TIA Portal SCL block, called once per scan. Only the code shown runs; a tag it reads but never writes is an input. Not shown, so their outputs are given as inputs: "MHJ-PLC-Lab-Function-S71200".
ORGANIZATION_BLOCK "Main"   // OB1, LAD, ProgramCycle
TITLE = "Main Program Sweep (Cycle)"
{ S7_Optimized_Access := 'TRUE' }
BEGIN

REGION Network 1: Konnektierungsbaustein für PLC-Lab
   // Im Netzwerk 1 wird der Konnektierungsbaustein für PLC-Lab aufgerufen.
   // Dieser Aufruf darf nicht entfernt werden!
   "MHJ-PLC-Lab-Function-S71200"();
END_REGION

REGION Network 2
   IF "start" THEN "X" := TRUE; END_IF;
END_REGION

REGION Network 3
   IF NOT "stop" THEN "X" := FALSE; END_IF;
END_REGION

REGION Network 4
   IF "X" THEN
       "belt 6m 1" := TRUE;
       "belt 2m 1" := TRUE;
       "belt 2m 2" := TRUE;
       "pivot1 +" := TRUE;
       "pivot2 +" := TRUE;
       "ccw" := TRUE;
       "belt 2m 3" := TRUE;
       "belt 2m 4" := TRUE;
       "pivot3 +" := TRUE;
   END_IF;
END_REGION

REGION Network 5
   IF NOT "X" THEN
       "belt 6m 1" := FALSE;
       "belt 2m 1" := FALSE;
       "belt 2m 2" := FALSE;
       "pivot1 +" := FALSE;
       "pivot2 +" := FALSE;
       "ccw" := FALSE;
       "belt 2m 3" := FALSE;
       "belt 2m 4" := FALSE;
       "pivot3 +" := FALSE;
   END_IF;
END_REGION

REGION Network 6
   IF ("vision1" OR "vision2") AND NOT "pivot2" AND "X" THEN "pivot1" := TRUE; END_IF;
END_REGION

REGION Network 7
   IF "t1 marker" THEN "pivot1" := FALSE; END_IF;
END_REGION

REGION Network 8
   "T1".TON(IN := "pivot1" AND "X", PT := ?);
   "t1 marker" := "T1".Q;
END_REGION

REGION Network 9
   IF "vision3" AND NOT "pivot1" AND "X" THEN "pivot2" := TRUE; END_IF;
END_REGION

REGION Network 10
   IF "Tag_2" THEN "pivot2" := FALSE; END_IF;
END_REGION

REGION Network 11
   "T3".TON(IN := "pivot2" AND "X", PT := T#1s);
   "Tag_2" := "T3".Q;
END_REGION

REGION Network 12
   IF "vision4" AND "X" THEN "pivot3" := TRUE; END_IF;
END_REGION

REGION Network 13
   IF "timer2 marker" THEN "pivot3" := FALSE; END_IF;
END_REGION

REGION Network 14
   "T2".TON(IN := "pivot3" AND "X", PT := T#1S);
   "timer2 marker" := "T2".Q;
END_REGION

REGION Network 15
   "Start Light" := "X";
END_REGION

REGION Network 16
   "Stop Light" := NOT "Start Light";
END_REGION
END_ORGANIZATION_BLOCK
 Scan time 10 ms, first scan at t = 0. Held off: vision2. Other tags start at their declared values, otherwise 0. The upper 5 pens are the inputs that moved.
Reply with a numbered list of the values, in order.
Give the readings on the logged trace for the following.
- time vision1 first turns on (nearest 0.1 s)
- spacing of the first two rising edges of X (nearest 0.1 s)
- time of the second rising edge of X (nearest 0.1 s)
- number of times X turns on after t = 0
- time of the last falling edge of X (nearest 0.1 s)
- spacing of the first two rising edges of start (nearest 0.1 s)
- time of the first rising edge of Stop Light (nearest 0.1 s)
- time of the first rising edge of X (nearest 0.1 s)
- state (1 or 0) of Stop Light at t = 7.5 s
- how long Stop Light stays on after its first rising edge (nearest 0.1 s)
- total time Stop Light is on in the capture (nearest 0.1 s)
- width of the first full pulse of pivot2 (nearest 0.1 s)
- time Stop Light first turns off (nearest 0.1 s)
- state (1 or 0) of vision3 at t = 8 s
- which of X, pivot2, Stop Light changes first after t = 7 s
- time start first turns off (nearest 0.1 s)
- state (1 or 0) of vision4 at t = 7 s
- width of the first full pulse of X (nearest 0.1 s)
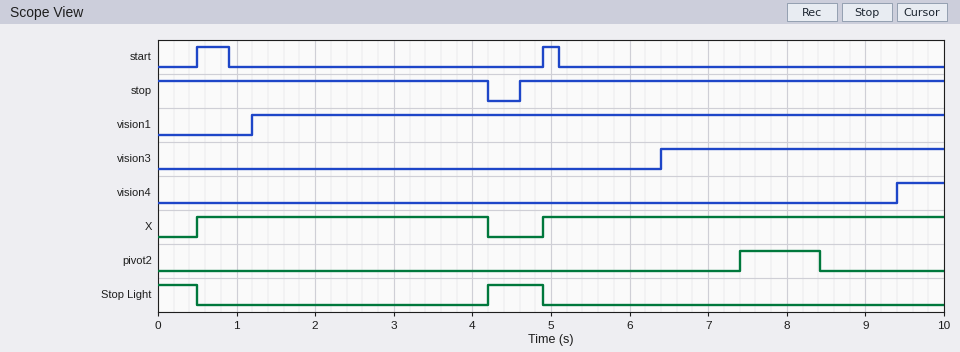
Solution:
1. 1.2 s
2. 4.4 s
3. 4.9 s
4. 2
5. 4.2 s
6. 4.4 s
7. 4.2 s
8. 0.5 s
9. 0
10. 0.7 s
11. 1.2 s
12. 1.0 s
13. 0.5 s
14. 1
15. pivot2
16. 0.9 s
17. 0
18. 3.7 s
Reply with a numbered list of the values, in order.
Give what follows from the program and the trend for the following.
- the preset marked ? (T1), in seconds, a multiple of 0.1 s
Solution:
1. 2.5 s
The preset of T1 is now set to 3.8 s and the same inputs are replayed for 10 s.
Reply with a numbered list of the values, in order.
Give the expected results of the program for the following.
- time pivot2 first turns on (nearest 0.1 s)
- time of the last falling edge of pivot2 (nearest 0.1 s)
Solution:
1. 8.7 s
2. 9.7 s
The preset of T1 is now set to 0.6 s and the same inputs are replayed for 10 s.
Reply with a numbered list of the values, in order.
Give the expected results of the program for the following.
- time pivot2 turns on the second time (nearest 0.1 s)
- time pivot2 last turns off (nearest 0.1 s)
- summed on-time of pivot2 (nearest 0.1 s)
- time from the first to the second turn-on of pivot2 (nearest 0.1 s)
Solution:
1. 8.4 s
2. 9.4 s
3. 2.0 s
4. 1.6 s
